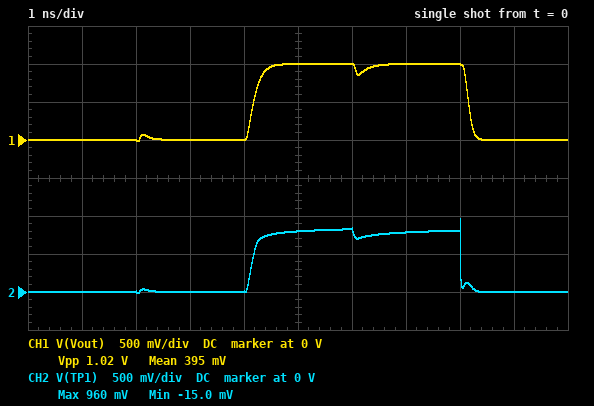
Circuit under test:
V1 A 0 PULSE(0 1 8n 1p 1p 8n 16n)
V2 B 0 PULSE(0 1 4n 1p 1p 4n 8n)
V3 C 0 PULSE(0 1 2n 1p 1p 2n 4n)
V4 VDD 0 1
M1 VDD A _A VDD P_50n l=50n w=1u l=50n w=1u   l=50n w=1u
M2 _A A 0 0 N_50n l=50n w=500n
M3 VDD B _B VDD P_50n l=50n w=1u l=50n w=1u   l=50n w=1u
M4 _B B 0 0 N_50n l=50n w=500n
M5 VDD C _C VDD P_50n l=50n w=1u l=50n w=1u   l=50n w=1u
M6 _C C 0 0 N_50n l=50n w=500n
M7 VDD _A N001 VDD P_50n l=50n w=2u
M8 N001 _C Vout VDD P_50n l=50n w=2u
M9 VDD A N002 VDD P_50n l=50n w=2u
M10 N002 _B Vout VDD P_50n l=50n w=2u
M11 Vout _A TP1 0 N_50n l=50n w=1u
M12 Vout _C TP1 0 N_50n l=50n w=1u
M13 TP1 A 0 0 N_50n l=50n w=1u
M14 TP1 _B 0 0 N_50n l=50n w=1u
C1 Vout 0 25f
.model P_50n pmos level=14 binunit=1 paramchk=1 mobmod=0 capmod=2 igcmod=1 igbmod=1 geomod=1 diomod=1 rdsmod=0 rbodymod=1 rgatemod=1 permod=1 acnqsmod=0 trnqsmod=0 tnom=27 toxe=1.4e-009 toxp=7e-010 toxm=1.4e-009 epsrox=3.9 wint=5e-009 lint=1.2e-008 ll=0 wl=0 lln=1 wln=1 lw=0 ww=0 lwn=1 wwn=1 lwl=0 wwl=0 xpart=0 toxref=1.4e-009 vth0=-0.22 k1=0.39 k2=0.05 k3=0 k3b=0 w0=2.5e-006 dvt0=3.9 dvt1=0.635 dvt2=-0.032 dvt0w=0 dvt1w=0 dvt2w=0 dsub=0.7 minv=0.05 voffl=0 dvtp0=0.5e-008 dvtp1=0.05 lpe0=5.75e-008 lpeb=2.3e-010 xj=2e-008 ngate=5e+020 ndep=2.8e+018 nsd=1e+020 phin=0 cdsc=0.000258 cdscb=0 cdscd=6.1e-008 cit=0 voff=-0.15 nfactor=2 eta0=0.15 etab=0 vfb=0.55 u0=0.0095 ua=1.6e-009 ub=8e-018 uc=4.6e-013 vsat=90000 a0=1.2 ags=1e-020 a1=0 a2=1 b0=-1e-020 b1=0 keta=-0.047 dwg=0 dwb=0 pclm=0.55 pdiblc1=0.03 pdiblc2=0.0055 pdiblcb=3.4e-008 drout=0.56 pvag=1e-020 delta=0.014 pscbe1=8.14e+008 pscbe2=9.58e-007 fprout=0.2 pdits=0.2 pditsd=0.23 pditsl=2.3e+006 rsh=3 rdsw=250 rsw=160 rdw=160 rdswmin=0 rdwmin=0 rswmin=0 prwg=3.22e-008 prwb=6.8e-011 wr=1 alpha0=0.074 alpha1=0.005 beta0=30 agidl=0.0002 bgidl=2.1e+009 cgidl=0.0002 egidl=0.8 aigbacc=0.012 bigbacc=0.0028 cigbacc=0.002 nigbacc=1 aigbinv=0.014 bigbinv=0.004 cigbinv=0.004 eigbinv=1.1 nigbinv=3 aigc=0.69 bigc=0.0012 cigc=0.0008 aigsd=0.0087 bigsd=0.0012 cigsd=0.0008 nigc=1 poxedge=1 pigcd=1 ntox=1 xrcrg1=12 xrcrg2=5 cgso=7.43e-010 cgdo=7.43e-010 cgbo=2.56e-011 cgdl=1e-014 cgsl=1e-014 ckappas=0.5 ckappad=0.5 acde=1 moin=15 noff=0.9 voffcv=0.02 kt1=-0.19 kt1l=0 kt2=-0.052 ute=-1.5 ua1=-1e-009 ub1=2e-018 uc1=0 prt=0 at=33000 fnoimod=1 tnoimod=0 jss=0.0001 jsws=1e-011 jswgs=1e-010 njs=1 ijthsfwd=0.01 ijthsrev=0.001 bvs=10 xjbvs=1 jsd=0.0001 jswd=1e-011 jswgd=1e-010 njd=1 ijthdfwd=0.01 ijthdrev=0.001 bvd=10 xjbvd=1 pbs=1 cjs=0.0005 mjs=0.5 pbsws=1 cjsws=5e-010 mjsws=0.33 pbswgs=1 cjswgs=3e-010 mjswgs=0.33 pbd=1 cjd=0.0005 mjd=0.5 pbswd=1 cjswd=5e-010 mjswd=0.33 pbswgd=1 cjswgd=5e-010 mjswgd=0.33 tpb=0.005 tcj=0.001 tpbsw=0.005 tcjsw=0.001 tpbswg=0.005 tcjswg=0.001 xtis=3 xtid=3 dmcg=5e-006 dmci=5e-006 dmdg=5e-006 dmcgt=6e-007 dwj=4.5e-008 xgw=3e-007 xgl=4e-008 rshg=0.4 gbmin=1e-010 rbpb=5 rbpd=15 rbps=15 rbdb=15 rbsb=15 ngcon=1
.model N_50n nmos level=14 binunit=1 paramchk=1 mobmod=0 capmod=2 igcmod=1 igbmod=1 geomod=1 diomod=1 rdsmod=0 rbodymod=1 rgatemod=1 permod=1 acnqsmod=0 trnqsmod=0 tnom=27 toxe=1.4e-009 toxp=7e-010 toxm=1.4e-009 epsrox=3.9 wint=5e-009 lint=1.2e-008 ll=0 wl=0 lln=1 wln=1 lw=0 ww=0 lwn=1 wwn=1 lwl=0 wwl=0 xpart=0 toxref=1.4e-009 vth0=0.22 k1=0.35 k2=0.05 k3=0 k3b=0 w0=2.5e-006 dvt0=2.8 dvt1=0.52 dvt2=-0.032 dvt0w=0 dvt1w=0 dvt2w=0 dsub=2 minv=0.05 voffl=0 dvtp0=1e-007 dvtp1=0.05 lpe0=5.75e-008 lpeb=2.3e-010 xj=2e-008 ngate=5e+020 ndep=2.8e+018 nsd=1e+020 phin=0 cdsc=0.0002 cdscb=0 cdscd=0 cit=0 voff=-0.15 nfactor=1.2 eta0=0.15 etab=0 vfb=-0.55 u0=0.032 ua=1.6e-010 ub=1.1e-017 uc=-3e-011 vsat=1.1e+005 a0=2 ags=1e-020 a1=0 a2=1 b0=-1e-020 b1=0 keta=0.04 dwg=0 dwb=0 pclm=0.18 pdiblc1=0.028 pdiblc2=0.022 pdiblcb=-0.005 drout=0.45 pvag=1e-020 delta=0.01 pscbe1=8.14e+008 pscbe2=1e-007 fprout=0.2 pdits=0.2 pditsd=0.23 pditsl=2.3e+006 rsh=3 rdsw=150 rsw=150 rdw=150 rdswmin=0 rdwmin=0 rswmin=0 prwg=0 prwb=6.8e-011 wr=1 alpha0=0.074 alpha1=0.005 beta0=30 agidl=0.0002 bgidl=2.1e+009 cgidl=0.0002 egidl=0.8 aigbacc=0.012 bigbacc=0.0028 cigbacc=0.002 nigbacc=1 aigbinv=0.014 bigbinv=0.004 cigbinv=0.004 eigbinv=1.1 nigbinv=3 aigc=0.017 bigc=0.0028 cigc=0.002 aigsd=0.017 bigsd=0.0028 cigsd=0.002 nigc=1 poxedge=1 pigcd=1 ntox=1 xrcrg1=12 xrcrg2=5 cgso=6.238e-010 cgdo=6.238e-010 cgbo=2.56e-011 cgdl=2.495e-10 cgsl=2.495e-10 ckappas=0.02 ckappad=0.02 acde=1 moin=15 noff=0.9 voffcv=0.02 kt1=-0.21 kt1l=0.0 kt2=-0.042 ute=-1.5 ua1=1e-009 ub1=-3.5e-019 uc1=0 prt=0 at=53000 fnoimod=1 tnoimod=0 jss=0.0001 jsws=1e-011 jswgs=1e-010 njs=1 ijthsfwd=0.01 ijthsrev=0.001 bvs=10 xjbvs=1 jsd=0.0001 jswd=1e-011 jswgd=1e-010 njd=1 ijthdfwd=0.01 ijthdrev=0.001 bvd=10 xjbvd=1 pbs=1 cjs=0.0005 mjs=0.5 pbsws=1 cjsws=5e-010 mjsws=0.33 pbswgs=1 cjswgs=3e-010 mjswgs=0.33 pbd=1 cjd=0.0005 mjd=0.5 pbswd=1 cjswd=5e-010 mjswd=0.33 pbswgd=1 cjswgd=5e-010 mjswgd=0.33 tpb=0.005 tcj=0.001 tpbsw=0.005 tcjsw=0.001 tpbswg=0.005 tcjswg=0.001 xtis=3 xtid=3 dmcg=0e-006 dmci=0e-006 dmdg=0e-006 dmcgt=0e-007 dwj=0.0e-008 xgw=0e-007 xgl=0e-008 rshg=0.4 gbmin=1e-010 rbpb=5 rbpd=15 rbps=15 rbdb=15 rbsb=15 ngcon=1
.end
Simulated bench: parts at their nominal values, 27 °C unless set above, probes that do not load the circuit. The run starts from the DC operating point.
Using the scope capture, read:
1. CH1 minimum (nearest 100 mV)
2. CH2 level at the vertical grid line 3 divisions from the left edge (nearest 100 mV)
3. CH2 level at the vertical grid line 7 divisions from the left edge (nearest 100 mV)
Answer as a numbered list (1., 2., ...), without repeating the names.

1. 0 V
2. 0 V
3. 800 mV
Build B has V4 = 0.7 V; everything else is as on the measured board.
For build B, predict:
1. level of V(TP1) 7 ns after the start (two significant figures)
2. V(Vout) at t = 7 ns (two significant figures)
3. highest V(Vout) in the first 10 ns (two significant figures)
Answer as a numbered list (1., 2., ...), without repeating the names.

1. 510 mV
2. 700 mV
3. 710 mV
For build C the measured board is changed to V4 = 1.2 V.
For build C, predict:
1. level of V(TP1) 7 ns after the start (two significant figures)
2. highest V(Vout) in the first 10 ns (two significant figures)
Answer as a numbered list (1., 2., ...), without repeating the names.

1. 970 mV
2. 1.2 V
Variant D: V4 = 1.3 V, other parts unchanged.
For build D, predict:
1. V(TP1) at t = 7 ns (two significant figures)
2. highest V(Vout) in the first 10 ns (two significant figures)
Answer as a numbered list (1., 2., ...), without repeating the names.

1. 1.1 V
2. 1.3 V
